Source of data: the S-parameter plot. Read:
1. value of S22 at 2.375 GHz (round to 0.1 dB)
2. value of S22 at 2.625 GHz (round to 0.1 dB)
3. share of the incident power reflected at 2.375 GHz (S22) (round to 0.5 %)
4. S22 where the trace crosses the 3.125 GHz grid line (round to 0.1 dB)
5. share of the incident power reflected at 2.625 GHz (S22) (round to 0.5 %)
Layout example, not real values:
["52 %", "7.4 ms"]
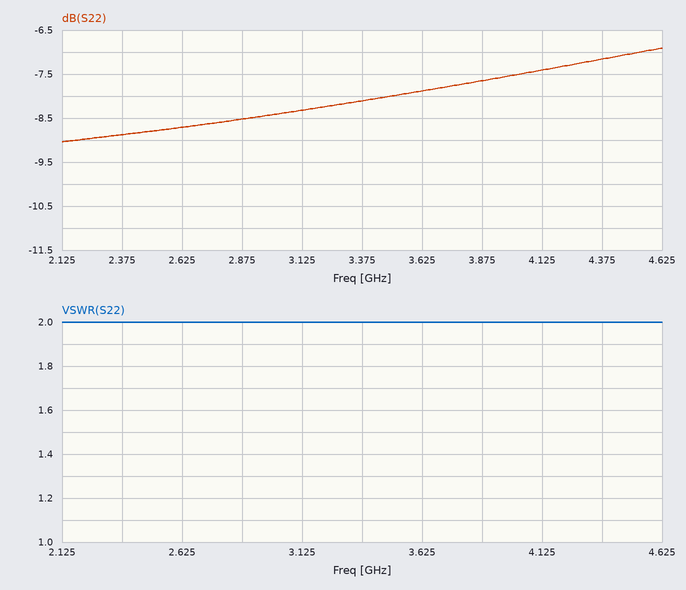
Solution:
["-8.9 dB", "-8.7 dB", "13.0 %", "-8.3 dB", "13.5 %"]
